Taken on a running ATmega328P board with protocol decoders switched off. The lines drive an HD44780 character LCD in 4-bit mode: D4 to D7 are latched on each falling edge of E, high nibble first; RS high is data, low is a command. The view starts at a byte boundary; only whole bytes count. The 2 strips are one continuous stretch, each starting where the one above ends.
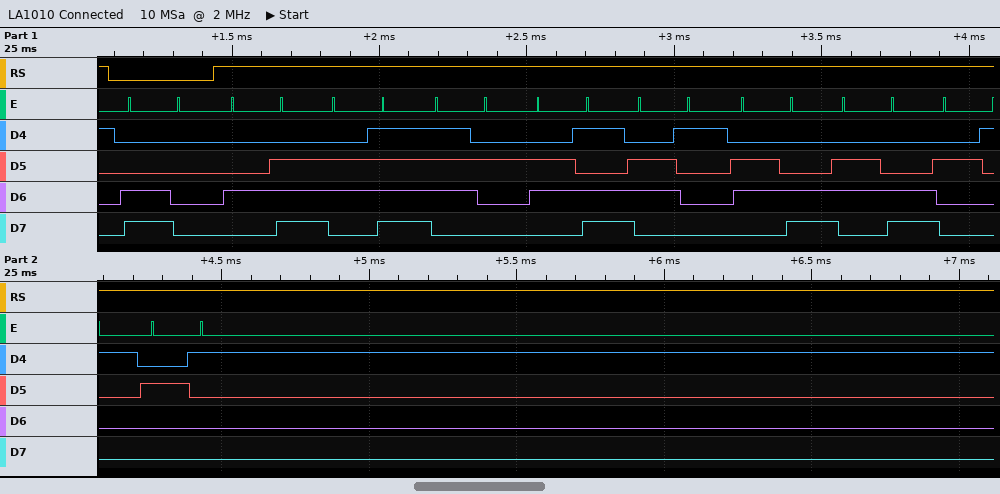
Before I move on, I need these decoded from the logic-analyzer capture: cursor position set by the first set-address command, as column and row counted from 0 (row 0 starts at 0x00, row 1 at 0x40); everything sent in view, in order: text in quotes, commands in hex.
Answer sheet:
column 0, row 1
0xC0 "Normall!!"
